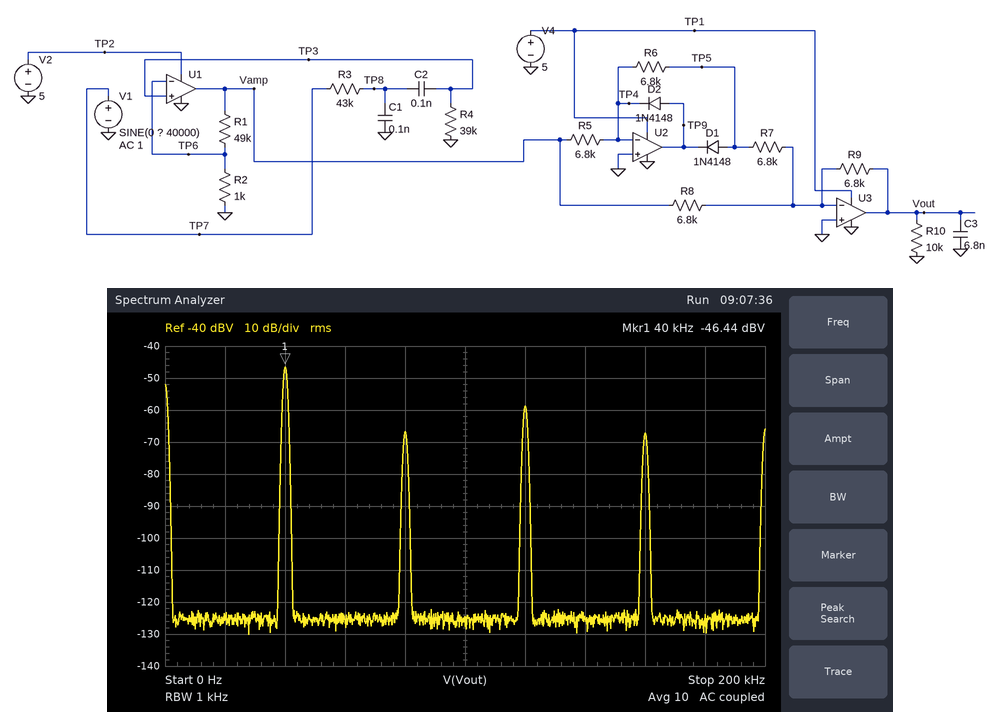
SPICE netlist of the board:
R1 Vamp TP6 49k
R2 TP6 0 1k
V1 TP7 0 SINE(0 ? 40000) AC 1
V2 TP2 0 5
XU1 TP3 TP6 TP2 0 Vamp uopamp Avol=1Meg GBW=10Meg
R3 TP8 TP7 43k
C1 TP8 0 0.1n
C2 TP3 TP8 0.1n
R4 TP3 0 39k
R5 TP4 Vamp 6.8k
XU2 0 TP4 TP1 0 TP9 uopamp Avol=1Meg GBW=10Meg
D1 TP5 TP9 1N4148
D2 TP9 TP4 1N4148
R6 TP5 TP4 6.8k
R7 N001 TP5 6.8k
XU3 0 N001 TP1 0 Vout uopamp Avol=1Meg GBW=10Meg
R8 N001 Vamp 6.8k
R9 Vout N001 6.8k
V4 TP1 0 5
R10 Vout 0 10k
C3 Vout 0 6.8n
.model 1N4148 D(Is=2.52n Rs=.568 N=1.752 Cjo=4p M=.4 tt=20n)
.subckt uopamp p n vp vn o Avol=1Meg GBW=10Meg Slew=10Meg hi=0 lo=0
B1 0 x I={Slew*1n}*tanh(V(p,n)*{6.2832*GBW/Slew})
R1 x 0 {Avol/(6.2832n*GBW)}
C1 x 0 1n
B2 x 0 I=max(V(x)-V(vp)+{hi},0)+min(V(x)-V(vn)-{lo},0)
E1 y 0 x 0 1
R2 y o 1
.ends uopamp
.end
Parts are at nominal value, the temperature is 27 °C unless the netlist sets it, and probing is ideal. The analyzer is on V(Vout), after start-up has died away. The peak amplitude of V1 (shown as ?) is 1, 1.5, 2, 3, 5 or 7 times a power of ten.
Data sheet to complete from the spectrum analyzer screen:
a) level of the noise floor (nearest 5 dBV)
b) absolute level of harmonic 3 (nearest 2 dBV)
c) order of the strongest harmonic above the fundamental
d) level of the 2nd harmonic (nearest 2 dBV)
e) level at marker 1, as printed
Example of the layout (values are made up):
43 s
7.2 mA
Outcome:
-125 dBV
-58 dBV
3
-66 dBV
-46.44 dBV
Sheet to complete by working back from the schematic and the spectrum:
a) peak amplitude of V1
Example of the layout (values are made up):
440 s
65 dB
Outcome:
70 mV
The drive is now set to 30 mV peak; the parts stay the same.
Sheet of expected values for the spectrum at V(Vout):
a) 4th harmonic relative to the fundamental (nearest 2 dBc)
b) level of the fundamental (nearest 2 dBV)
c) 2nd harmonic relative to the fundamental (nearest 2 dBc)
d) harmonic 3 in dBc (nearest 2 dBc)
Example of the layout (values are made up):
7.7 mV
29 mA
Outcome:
-18 dBc
-48 dBV
-12 dBc
-18 dBc
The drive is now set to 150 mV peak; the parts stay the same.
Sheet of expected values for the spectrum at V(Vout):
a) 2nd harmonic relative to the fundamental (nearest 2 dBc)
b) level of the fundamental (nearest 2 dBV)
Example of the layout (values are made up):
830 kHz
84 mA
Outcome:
-28 dBc
-46 dBV
